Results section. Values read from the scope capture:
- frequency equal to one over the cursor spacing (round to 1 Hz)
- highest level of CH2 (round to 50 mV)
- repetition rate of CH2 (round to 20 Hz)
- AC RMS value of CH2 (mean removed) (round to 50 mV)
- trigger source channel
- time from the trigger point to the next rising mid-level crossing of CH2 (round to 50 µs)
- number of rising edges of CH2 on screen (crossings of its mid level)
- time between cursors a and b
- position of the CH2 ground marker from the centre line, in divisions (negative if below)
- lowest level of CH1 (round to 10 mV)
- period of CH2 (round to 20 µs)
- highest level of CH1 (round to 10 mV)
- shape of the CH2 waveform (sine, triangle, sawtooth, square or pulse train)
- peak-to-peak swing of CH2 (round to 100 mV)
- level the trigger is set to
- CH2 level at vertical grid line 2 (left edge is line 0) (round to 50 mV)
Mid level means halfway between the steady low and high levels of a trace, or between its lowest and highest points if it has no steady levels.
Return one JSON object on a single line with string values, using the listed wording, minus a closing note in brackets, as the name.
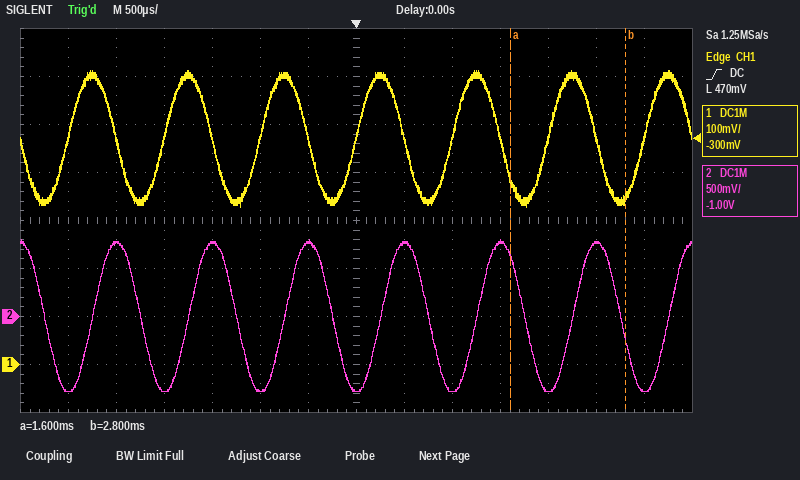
{"frequency equal to one over the cursor spacing": "833 Hz", "highest level of CH2": "800 mV", "repetition rate of CH2": "1.00 kHz", "AC RMS value of CH2 (mean removed)": "550 mV", "trigger source channel": "CH1", "time from the trigger point to the next rising mid-level crossing of CH2": "250 µs", "number of rising edges of CH2 on screen": "7", "time between cursors a and b": "1.20 ms", "position of the CH2 ground marker from the centre line, in divisions": "-2.0 div", "lowest level of CH1": "330 mV", "period of CH2": "1.00 ms", "highest level of CH1": "610 mV", "shape of the CH2 waveform": "sine", "peak-to-peak swing of CH2": "1.60 V", "level the trigger is set to": "470 mV", "CH2 level at vertical grid line 2 (left edge is line 0)": "750 mV"}
